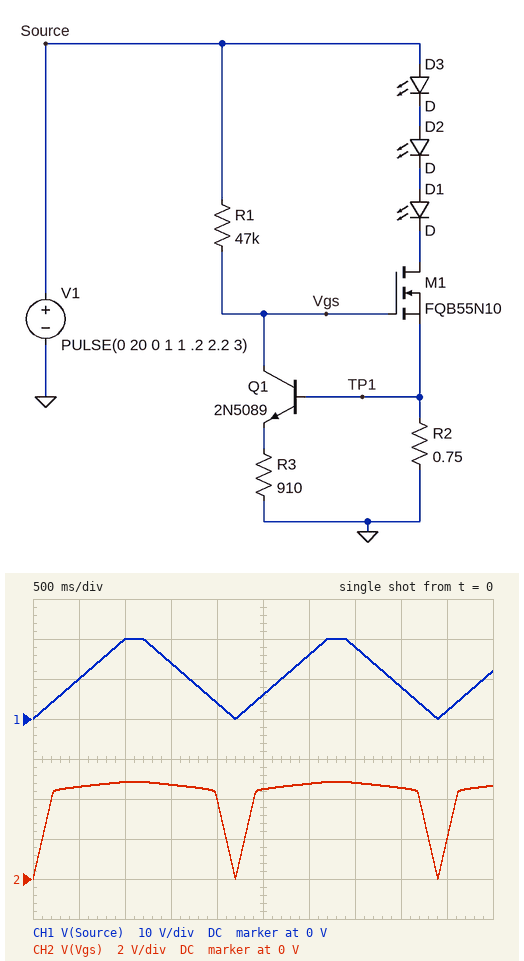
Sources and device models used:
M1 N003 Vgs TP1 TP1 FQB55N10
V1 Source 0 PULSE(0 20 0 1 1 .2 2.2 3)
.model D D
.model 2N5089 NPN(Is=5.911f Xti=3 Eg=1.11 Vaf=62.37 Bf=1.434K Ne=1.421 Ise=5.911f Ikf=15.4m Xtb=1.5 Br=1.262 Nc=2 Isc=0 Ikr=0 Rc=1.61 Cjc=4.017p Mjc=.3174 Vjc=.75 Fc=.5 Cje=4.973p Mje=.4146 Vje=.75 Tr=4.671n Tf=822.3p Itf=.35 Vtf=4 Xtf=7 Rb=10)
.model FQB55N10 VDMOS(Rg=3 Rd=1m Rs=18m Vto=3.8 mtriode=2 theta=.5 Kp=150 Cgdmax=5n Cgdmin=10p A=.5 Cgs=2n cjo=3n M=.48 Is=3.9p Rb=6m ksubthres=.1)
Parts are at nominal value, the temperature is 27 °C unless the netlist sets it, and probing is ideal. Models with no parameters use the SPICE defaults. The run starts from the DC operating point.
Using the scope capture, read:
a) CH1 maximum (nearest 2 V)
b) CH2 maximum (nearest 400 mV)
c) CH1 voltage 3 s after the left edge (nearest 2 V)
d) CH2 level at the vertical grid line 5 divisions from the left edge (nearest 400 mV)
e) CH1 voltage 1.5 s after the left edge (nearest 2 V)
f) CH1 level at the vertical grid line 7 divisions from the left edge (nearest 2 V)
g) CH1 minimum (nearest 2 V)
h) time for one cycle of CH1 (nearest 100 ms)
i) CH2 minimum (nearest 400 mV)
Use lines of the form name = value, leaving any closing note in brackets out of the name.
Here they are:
CH1 maximum = 20 V
CH2 maximum = 4.8 V
CH1 voltage 3 s after the left edge = 16 V
CH2 level at the vertical grid line 5 divisions from the left edge = 4.4 V
CH1 voltage 1.5 s after the left edge = 14 V
CH1 level at the vertical grid line 7 divisions from the left edge = 18 V
CH1 minimum = 0 V
time for one cycle of CH1 = 2.2 s
CH2 minimum = 0 V
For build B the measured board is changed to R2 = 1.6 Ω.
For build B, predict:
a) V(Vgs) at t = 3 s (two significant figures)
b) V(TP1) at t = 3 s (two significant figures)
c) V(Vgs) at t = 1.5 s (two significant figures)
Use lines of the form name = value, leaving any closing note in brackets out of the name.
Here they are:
V(Vgs) at t = 3 s = 4.7 V
V(TP1) at t = 3 s = 850 mV
V(Vgs) at t = 1.5 s = 4.6 V
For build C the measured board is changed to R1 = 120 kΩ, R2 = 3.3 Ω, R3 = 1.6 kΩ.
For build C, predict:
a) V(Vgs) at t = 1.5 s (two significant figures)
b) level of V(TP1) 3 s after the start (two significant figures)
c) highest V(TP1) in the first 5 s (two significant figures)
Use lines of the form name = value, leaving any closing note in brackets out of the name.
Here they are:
V(Vgs) at t = 1.5 s = 4.5 V
level of V(TP1) 3 s after the start = 760 mV
highest V(TP1) in the first 5 s = 820 mV
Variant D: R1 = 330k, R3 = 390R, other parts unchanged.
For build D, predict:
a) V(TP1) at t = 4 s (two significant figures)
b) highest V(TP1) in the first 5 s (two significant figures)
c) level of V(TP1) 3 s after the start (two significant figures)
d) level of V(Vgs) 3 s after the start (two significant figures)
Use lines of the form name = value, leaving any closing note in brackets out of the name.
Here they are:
V(TP1) at t = 4 s = 550 mV
highest V(TP1) in the first 5 s = 610 mV
level of V(TP1) 3 s after the start = 590 mV
level of V(Vgs) 3 s after the start = 4.5 V
